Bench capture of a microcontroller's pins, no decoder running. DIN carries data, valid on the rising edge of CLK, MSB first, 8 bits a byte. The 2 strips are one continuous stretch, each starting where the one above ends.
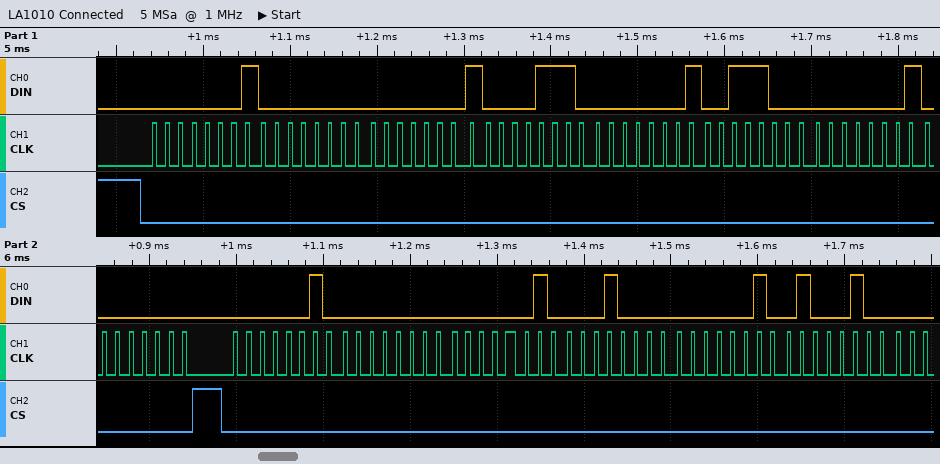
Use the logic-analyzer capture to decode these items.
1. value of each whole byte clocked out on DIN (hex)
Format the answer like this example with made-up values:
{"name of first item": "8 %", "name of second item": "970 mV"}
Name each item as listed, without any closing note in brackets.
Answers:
{"value of each whole byte clocked out on DIN": "01 00 01 0E 01 38 01 00 02 00 02 10 02 44"}
